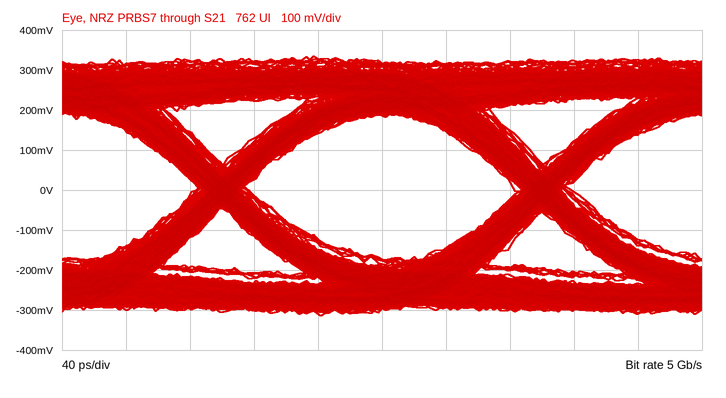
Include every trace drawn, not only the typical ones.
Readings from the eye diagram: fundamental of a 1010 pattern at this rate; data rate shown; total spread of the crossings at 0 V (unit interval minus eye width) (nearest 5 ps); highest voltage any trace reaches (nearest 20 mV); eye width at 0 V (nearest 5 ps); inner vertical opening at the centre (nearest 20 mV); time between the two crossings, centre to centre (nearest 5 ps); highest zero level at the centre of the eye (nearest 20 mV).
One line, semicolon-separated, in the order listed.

2.5 GHz; 5 Gb/s; 35 ps; 340 mV; 165 ps; 360 mV; 200 ps; -180 mV
